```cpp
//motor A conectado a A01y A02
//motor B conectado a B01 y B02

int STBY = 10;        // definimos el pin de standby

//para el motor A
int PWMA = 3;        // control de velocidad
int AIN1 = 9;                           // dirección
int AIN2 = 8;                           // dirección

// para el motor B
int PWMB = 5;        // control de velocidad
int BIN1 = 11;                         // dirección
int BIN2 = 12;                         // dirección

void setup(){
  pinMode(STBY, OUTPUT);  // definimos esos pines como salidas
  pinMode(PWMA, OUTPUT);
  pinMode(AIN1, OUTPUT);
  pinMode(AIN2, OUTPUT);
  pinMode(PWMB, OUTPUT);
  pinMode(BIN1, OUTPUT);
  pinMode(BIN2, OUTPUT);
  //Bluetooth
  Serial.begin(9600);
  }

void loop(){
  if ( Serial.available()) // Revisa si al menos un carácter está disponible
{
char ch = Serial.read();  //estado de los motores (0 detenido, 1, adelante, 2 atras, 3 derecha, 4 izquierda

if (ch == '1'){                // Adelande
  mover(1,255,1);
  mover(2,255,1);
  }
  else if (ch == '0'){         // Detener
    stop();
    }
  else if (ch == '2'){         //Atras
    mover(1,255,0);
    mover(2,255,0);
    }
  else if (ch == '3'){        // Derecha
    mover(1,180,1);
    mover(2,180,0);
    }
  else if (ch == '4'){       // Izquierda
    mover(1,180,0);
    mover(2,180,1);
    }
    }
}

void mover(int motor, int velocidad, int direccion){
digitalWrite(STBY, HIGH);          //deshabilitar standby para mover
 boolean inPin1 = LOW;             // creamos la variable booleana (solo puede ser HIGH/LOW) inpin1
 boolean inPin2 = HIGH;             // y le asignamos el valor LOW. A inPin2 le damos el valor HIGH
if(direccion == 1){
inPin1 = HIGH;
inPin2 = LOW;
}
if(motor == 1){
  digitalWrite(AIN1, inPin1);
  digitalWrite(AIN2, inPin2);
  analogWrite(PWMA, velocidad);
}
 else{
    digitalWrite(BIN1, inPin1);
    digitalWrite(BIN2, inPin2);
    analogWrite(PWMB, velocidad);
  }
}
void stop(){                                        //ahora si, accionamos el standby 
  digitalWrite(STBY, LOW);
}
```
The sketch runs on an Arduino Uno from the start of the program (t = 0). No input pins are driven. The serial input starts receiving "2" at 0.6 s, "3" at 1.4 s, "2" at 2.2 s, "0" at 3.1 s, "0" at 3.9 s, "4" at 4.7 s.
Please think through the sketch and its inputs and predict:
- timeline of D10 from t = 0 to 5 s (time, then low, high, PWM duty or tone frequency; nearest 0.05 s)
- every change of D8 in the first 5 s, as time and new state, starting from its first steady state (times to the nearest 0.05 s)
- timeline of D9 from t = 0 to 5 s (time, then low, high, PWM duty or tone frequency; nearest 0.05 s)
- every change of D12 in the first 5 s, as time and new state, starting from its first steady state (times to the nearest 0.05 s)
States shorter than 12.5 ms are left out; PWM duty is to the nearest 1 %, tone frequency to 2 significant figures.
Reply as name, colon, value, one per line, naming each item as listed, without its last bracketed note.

timeline of D10 from t = 0 to 5 s: 0 s low; 0.6 s high; 3.1 s low; 4.7 s high
every change of D8 in the first 5 s, as time and new state, starting from its first steady state: 0 s low; 0.6 s high; 1.4 s low; 2.2 s high
timeline of D9 from t = 0 to 5 s: 0 s low; 1.4 s high; 2.2 s low
every change of D12 in the first 5 s, as time and new state, starting from its first steady state: 0 s low; 0.6 s high; 4.7 s low
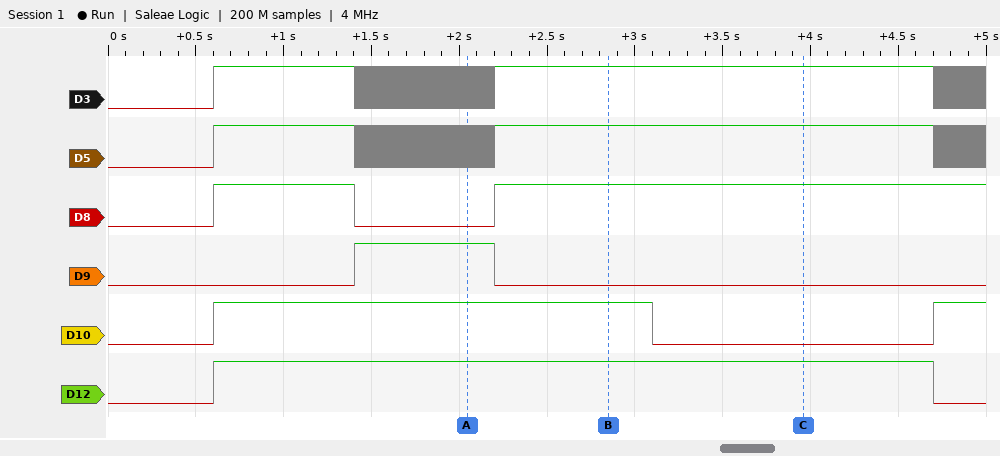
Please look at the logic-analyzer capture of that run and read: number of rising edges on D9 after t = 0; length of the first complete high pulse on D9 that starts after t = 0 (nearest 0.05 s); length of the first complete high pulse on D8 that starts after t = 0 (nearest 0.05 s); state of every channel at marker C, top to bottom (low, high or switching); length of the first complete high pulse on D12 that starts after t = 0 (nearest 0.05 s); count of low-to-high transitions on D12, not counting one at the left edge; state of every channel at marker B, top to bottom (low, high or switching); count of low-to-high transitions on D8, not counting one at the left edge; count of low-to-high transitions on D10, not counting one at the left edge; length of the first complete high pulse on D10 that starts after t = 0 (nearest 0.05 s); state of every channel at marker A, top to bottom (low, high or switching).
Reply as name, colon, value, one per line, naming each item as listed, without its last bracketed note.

number of rising edges on D9 after t = 0: 1
length of the first complete high pulse on D9 that starts after t = 0: 0.80 s
length of the first complete high pulse on D8 that starts after t = 0: 0.80 s
state of every channel at marker C, top to bottom: D3 high, D5 high, D8 high, D9 low, D10 low, D12 high
length of the first complete high pulse on D12 that starts after t = 0: 4.10 s
count of low-to-high transitions on D12, not counting one at the left edge: 1
state of every channel at marker B, top to bottom: D3 high, D5 high, D8 high, D9 low, D10 high, D12 high
count of low-to-high transitions on D8, not counting one at the left edge: 2
count of low-to-high transitions on D10, not counting one at the left edge: 2
length of the first complete high pulse on D10 that starts after t = 0: 2.50 s
state of every channel at marker A, top to bottom: D3 switching, D5 switching, D8 low, D9 high, D10 high, D12 high
